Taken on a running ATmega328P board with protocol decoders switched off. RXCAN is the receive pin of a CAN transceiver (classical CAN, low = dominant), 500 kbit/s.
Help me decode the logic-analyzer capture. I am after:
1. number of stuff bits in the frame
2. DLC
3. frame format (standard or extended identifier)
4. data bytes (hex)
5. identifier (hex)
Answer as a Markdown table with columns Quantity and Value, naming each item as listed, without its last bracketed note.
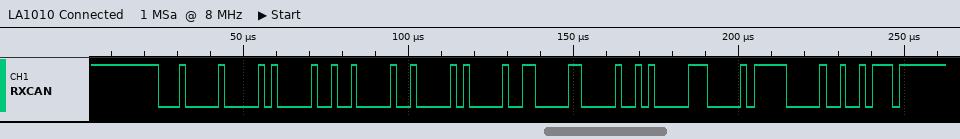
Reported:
| Quantity | Value |
|---|---|
| number of stuff bits in the frame | 12 |
| DLC | 8 |
| frame format | standard |
| data bytes | 09 01 02 03 04 05 06 07 |
| identifier | 0x100 |
